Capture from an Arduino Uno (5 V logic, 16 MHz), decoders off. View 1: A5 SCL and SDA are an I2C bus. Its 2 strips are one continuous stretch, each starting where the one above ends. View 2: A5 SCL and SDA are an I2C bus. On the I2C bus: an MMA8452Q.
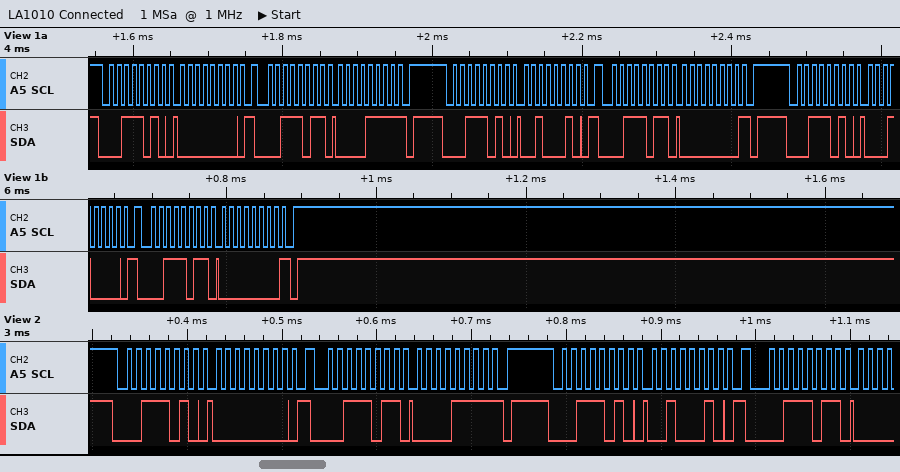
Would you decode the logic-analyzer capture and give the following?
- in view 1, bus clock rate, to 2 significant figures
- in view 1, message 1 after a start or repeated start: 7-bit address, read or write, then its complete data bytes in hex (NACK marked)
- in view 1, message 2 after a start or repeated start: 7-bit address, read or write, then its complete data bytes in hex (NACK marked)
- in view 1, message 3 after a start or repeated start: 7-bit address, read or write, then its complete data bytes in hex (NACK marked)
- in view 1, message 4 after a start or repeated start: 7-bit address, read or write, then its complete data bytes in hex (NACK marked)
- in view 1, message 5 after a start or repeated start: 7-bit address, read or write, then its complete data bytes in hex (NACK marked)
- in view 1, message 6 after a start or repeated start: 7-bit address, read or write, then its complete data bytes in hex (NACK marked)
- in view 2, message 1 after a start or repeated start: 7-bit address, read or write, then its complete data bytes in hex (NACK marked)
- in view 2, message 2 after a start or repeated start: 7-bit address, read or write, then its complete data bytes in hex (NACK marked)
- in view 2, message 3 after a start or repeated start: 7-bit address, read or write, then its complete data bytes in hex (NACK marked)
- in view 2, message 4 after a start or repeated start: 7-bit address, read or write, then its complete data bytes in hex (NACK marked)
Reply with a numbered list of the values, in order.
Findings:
1. 100 kHz
2. 0x1D write: 00
3. 0x1D read: 0F NACK
4. 0x1D write: 22
5. 0x1D read: 00 NACK
6. 0x1D write: 10
7. 0x1D read: 00 NACK
8. 0x1D write: 00
9. 0x1D read: 0F NACK
10. 0x1D write: 22
11. 0x1D read
